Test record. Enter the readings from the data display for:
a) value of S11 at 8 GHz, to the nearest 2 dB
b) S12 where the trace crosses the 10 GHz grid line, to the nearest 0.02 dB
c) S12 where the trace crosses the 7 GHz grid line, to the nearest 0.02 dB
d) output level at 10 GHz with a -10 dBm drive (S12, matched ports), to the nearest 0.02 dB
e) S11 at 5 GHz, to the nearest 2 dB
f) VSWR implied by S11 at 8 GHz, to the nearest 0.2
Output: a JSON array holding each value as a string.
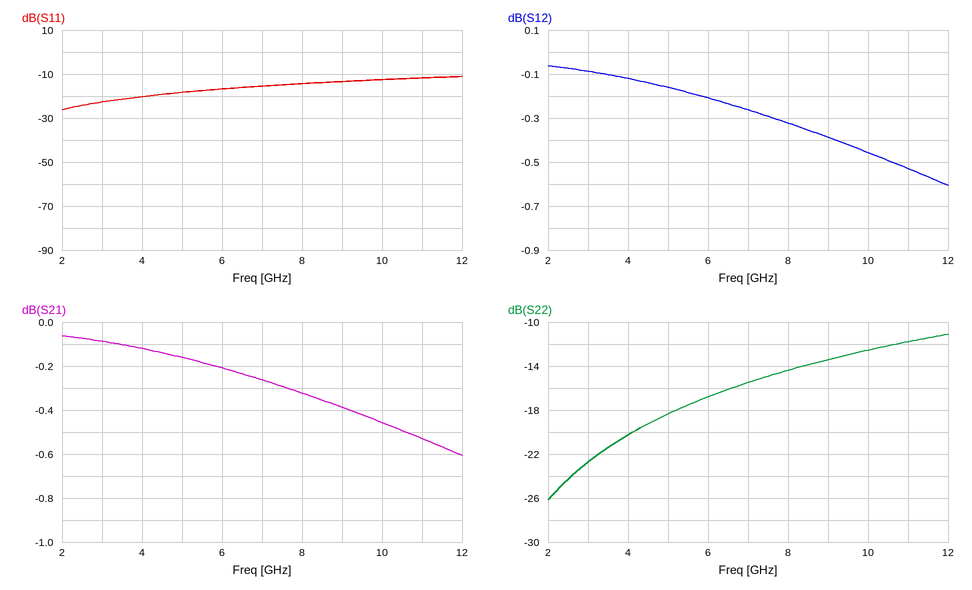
["-14 dB", "-0.46 dB", "-0.26 dB", "-10.46 dBm", "-18 dB", "1.4"]
